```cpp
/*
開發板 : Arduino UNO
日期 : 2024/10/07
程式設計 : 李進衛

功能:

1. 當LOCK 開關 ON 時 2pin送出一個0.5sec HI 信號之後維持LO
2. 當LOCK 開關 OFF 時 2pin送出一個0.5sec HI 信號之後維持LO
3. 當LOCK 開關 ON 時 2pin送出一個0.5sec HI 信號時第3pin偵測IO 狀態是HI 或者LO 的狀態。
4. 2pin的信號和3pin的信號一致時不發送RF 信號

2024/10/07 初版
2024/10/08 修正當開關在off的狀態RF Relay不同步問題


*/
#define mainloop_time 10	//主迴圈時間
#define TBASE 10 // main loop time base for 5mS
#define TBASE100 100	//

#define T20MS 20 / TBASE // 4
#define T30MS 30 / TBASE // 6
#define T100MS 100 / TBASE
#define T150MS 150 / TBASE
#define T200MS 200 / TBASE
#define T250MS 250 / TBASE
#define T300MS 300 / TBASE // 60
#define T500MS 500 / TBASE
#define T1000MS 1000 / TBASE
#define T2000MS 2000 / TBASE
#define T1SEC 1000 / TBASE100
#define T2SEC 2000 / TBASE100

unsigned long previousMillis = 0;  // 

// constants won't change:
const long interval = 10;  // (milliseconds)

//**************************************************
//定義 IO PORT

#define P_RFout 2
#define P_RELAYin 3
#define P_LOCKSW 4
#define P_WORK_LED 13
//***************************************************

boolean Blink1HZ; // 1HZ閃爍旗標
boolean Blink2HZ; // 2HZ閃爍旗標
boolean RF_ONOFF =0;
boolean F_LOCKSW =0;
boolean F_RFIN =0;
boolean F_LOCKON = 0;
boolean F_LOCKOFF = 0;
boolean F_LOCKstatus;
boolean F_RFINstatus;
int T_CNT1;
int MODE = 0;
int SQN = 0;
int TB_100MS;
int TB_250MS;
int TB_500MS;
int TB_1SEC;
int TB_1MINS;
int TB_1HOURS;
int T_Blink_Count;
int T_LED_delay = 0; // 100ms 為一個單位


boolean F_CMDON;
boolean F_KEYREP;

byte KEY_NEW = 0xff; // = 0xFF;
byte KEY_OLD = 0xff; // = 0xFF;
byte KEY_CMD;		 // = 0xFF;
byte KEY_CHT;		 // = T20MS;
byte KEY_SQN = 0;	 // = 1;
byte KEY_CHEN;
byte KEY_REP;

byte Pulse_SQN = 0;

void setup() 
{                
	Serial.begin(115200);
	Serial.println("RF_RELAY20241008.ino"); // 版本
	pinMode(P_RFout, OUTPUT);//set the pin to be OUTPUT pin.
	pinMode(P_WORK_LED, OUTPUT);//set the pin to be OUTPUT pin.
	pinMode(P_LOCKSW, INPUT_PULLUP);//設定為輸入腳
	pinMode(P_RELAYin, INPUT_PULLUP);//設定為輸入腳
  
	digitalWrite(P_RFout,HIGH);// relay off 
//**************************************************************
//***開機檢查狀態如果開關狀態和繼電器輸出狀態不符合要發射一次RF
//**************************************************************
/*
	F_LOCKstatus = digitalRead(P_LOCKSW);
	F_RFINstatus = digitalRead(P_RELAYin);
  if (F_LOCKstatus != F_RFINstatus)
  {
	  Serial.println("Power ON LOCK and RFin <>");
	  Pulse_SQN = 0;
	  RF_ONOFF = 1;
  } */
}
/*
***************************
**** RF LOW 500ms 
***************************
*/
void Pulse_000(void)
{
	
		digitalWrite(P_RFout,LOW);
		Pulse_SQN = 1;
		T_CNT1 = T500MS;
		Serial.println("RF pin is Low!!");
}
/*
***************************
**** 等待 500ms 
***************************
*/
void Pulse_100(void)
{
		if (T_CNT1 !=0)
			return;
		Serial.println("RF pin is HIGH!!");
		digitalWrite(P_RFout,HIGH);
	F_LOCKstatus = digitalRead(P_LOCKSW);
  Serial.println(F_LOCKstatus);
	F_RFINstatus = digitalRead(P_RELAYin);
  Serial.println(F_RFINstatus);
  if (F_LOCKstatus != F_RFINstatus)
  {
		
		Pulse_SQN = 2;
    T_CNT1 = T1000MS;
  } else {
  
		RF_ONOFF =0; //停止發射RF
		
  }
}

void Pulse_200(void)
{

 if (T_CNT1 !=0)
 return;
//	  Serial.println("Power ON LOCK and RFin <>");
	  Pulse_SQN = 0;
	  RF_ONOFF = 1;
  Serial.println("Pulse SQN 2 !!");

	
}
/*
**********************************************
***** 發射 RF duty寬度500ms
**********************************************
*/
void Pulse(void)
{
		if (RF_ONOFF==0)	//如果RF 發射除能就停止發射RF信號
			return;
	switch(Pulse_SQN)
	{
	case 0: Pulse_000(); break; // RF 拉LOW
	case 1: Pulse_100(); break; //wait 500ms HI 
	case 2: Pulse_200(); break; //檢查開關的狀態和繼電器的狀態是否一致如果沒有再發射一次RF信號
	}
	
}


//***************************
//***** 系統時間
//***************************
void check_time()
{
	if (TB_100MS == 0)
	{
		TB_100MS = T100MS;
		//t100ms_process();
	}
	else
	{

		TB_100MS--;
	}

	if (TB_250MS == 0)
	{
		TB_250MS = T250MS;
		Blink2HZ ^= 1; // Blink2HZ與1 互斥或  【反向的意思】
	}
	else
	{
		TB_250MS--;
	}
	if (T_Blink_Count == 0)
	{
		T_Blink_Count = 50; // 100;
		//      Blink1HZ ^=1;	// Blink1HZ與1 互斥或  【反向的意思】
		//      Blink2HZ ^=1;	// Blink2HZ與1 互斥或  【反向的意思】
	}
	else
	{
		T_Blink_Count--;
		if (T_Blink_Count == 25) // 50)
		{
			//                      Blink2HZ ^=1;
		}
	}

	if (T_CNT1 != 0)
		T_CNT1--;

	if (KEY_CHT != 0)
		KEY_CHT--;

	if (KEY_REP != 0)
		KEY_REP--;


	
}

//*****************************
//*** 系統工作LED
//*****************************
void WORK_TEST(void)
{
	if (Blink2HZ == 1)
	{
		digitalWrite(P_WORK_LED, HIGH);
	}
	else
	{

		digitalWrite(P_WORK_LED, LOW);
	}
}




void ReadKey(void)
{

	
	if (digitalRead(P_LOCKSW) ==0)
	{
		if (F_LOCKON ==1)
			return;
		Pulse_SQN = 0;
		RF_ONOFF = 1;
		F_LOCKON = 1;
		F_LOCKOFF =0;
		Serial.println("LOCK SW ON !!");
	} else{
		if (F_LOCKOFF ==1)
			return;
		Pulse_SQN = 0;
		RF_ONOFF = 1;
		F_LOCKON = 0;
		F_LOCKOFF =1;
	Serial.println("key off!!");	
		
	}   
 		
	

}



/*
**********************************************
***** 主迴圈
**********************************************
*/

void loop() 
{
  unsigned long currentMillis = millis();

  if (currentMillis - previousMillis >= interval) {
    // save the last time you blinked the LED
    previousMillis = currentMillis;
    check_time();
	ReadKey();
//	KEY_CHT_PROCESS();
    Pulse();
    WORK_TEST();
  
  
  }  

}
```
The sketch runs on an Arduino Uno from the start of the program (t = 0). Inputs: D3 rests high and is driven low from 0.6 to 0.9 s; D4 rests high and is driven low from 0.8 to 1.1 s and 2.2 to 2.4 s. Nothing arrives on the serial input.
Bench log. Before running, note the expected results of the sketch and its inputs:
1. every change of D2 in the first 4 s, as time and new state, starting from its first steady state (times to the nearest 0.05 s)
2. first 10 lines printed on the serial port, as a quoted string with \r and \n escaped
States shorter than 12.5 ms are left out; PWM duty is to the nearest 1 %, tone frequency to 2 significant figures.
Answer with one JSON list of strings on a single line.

["0 s low; 0.5 s high; 0.8 s low; 1.6 s high; 2.2 s low; 2.9 s high", "\"RF_RELAY20241008.ino\\r\\nkey off!!\\r\\nRF pin is Low!!\\r\\nRF pin is HIGH!!\\r\\n1\\r\\n1\\r\\nLOCK SW ON !!\\r\\nRF pin is Low!!\\r\\nkey off!!\\r\\nRF pin is Low!!\\r\\n\""]
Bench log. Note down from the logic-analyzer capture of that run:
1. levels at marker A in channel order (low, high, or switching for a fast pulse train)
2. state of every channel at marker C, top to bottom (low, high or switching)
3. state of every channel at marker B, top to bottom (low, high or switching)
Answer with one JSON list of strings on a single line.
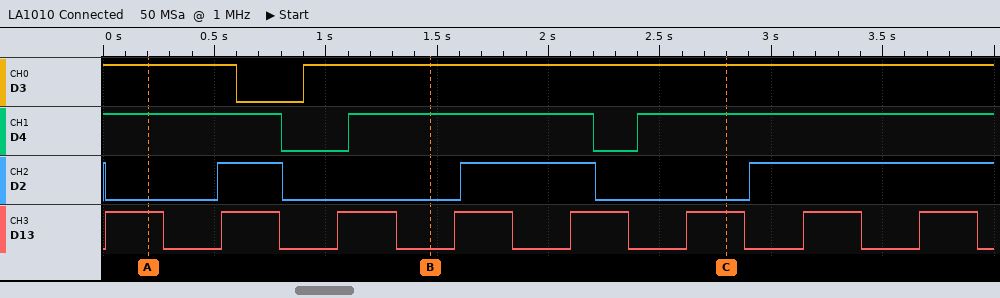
["D3 high, D4 high, D2 low, D13 high", "D3 high, D4 high, D2 low, D13 high", "D3 high, D4 high, D2 low, D13 low"]
